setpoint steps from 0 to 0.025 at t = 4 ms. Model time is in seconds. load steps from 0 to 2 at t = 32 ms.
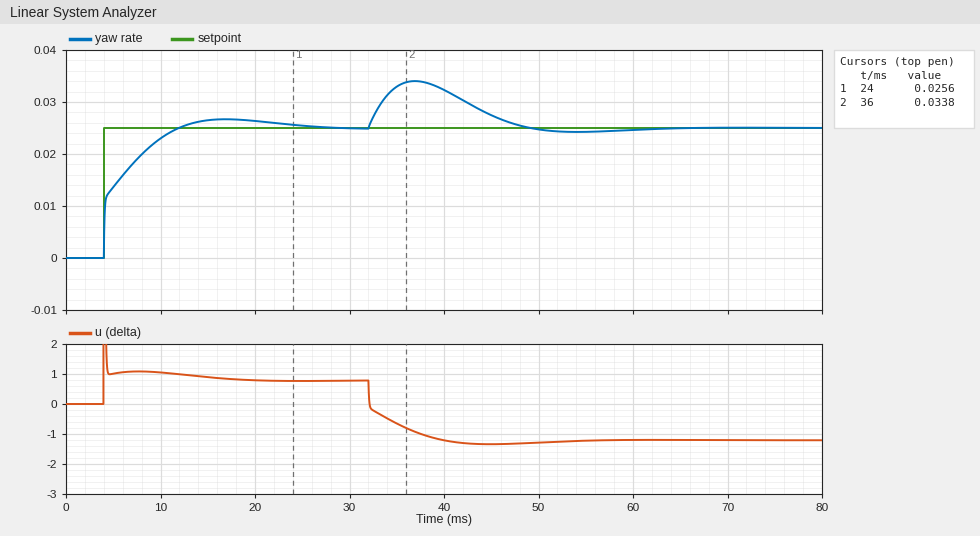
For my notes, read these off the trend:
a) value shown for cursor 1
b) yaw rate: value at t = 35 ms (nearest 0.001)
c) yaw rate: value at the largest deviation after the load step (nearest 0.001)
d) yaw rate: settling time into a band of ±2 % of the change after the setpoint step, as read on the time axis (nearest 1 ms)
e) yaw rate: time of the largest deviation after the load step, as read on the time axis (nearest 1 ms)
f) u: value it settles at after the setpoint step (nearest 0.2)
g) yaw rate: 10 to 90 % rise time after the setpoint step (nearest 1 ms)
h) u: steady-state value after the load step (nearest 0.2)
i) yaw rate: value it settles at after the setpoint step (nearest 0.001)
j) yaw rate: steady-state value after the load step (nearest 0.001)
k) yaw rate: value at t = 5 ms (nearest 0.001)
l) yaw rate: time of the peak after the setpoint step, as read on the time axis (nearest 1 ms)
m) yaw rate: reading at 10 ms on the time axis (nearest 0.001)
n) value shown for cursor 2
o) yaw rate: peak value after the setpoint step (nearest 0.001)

0.0256
0.033
0.034
25 ms
37 ms
0.8
6 ms
-1.2
0.025
0.025
0.014
17 ms
0.023
0.0338
0.027
